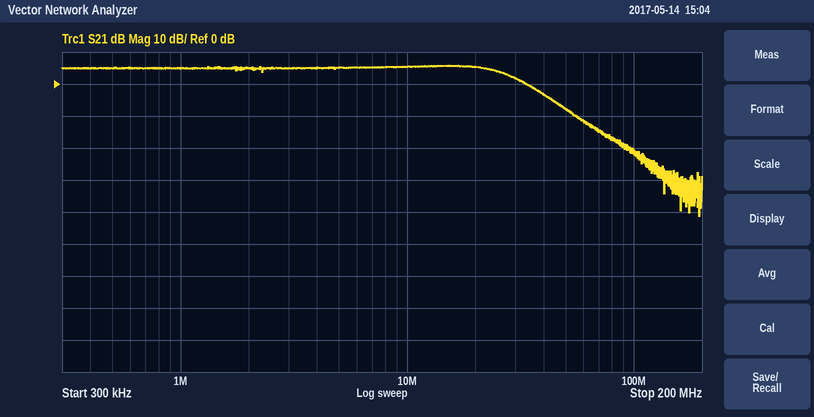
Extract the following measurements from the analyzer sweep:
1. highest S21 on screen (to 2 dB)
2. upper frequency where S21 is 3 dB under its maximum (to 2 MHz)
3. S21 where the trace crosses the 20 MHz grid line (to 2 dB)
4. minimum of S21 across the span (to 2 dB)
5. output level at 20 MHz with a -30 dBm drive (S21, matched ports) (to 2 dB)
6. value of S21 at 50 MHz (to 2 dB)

6 dB
28 MHz
6 dB
-42 dB
-24 dBm
-8 dB
